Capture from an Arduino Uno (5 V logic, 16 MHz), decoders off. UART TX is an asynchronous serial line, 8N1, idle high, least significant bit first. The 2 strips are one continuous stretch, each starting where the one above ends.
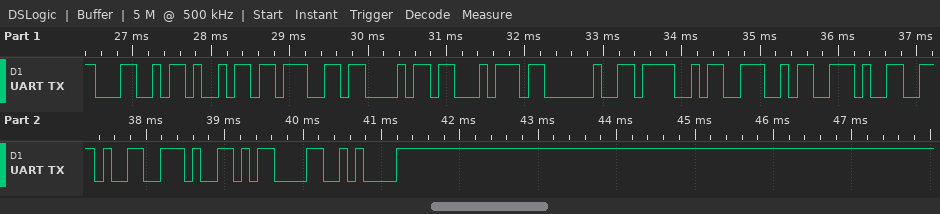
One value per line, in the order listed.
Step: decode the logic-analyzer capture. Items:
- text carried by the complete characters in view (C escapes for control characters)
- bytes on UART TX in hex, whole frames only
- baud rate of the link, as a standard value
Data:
"Light ON...\r\n"
0x4C 0x69 0x67 0x68 0x74 0x20 0x4F 0x4E 0x2E 0x2E 0x2E 0x0D 0x0A
9600 baud
